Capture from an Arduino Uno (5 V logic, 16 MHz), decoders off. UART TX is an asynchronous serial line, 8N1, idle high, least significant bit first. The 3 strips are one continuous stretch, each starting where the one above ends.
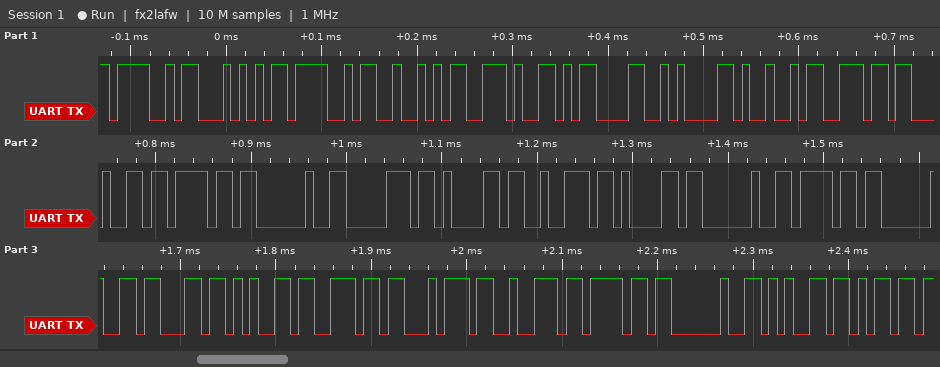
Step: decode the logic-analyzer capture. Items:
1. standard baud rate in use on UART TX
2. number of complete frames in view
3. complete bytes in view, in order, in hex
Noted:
115200 baud
28
4F 54 4F 52 2E 0D 0A 49 6E 64 6F 20 70 61 72 61 20 6F 20 63 65 6E 74 72 6F 20 65 6D
